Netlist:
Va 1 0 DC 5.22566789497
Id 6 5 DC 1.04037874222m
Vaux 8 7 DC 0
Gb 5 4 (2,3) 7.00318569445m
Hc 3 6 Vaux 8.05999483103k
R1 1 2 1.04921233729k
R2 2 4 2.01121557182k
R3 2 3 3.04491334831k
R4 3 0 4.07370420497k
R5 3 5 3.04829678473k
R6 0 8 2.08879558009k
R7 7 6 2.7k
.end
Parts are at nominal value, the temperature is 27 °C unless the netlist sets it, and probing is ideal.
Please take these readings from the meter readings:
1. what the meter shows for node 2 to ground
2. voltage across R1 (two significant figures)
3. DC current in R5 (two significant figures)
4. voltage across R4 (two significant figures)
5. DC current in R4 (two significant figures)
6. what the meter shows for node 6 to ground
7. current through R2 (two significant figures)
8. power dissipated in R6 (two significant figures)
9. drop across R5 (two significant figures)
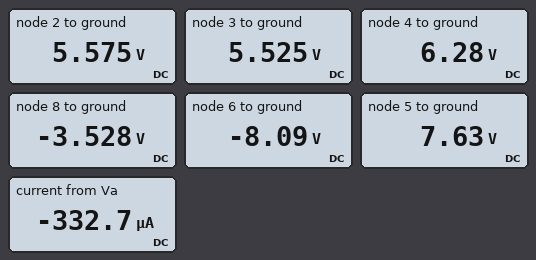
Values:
5.575 V
350 mV
690 µA
5.5 V
1.4 mA
-8.09 V
350 µA
6.0 mW
2.1 V
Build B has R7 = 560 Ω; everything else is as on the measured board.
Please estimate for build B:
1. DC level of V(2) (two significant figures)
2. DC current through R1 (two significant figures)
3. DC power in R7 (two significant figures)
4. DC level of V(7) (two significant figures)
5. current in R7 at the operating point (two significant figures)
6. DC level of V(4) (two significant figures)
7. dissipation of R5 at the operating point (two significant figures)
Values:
4.9 V
300 µA
470 µW
-1.9 V
920 µA
4.3 V
5.6 mW
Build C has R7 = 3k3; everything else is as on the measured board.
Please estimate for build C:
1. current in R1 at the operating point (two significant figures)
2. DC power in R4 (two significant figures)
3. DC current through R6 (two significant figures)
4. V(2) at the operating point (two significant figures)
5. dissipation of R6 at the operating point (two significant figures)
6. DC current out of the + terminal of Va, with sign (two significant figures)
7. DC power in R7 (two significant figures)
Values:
760 µA
8.6 mW
2.2 mA
6.0 V
10 mW
-760 µA
16 mW
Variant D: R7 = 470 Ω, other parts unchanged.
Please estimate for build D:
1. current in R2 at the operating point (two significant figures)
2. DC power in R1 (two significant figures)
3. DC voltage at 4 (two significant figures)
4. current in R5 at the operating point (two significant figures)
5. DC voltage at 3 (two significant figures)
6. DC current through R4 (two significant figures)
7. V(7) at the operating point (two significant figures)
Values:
330 µA
100 µW
4.2 V
1.4 mA
4.9 V
1.2 mA
-1.9 V
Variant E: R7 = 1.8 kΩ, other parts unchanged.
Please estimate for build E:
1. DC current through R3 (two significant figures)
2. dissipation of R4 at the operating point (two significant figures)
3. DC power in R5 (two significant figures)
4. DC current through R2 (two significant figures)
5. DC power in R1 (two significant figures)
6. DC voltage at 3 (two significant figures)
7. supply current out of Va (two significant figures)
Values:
1.5 µA
6.6 mW
3.5 mW
31 µA
930 nW
5.2 V
30 µA
